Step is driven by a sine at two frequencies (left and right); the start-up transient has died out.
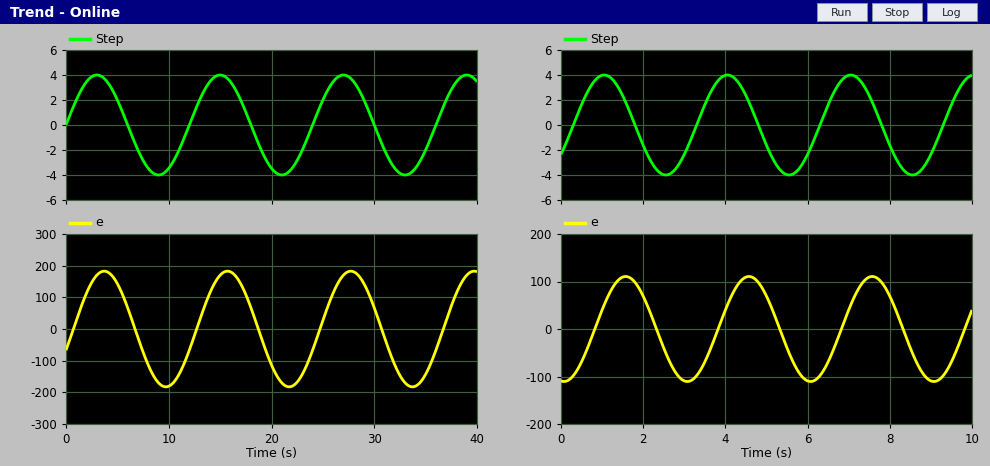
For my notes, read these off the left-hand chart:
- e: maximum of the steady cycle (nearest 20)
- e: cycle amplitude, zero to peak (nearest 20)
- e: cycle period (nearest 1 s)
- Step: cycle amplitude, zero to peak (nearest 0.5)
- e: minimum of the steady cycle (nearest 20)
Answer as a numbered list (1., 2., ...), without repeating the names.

1. 180
2. 180
3. 12 s
4. 4.0
5. -180
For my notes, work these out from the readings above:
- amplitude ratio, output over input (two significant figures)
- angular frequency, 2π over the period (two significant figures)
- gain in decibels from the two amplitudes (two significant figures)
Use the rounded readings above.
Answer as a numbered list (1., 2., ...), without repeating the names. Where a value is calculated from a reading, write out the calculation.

1. 180 / 4 = 45
2. 2π / 12 = 0.52 rad/s
3. 20 log10(180 / 4) = 33 dB
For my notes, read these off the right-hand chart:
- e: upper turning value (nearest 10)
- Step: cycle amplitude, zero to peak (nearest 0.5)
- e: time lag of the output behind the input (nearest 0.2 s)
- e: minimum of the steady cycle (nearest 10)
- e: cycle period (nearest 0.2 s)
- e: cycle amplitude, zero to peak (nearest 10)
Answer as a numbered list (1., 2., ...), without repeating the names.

1. 110
2. 4.0
3. 0.6 s
4. -110
5. 3.0 s
6. 110
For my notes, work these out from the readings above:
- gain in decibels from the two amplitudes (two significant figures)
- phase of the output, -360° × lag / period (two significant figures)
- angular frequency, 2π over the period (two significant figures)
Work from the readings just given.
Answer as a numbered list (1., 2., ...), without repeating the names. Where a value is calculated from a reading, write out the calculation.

1. 20 log10(110 / 4) = 29 dB
2. -360 × 0.6 / 3 = -72°
3. 2π / 3 = 2.1 rad/s
